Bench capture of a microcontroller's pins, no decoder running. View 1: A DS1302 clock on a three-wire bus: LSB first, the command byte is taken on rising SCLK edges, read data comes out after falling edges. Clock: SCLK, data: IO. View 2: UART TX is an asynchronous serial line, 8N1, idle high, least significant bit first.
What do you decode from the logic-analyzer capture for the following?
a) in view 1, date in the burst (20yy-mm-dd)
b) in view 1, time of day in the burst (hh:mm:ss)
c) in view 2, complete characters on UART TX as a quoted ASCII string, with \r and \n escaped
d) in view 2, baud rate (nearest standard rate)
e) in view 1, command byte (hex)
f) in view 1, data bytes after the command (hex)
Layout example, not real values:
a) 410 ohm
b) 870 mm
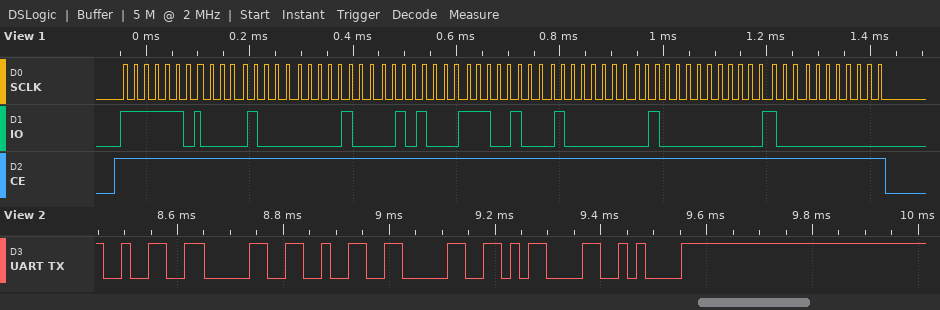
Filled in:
a) 2020-02-27
b) 14:20:10
c) "2020\r\n"
d) 57600 baud
e) 0xBF
f) 10 20 14 27 02 04 20 00
